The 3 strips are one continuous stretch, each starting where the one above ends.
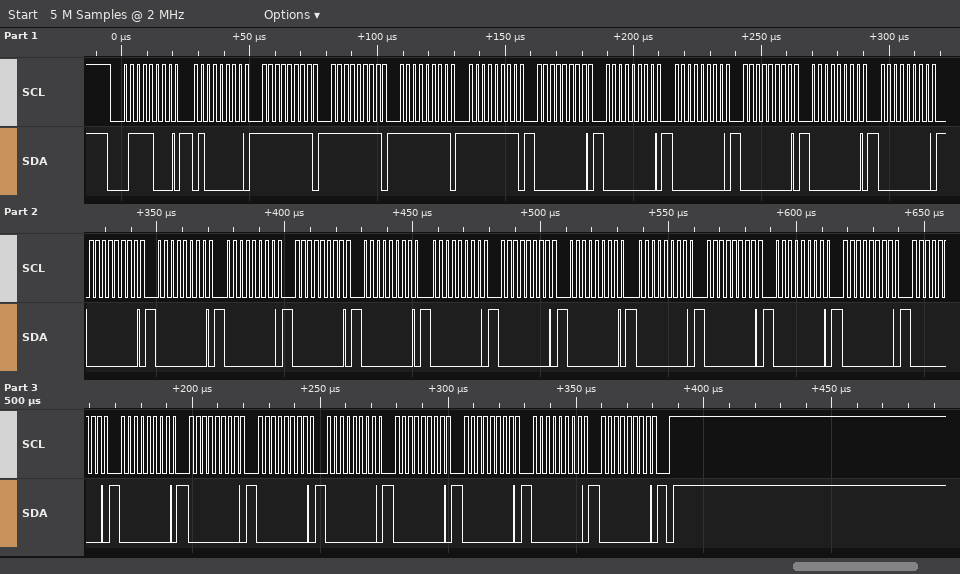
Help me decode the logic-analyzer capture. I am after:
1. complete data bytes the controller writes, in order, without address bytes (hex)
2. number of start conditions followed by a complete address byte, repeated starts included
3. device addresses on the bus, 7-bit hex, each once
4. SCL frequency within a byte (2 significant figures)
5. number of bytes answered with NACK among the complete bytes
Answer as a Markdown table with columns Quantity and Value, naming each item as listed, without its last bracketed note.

| Quantity | Value |
|---|---|
| complete data bytes the controller writes, in order, without address bytes | 40 FF FF FF FF 00 00 00 00 00 00 00 00 00 00 00 00 00 00 00 00 00 00 00 00 00 00 00 00 00 00 00 |
| number of start conditions followed by a complete address byte, repeated starts included | 1 |
| device addresses on the bus, 7-bit hex, each once | 0x3C |
| SCL frequency within a byte | 400 kHz |
| number of bytes answered with NACK among the complete bytes | 0 |
